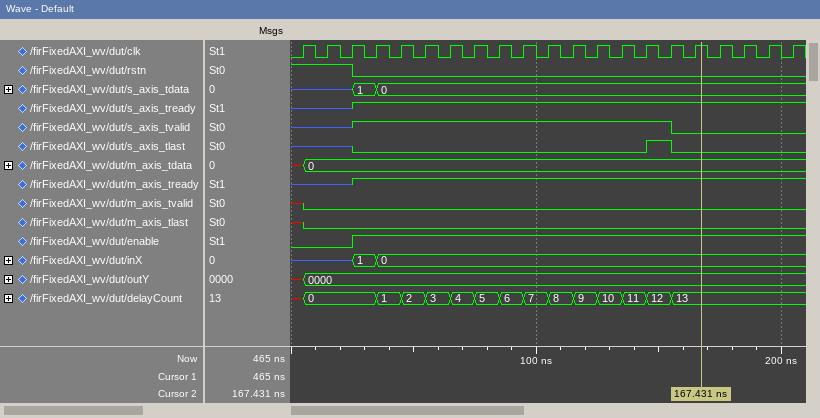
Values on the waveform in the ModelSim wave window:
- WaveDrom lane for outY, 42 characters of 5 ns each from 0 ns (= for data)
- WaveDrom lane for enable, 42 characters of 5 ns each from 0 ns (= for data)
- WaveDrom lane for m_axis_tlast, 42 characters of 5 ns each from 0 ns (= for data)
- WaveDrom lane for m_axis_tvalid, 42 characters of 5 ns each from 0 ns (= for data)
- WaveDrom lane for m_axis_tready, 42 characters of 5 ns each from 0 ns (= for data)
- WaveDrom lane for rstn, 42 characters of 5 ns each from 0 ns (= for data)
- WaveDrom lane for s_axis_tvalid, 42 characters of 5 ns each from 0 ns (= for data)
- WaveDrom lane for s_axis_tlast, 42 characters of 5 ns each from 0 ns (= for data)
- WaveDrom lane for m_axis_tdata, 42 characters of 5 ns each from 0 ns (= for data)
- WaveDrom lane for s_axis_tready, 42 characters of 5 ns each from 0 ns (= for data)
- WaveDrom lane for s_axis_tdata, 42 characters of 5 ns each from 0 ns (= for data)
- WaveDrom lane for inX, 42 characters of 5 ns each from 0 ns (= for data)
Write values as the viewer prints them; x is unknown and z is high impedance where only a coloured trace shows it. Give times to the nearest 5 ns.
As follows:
{name: 'outY', wave: 'x=........................................', data: '0000'}
{name: 'enable', wave: '0....1....................................'}
{name: 'm_axis_tlast', wave: 'x0........................................'}
{name: 'm_axis_tvalid', wave: 'x0........................................'}
{name: 'm_axis_tready', wave: 'z....1....................................'}
{name: 'rstn', wave: '1....0....................................'}
{name: 's_axis_tvalid', wave: 'z....1.........................0..........'}
{name: 's_axis_tlast', wave: 'z....0.......................1.0..........'}
{name: 'm_axis_tdata', wave: 'x=........................................', data: '0'}
{name: 's_axis_tready', wave: 'z....1....................................'}
{name: 's_axis_tdata', wave: 'z....=.=..................................', data: '1 0'}
{name: 'inX', wave: 'z....=.=..................................', data: '1 0'}
